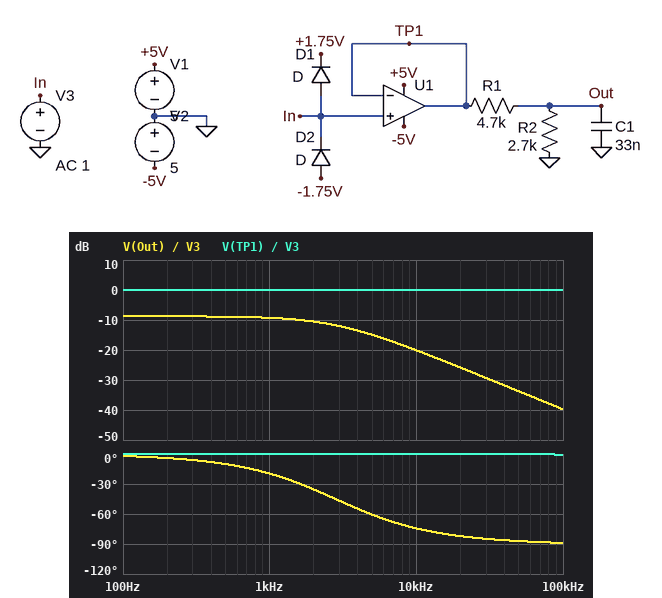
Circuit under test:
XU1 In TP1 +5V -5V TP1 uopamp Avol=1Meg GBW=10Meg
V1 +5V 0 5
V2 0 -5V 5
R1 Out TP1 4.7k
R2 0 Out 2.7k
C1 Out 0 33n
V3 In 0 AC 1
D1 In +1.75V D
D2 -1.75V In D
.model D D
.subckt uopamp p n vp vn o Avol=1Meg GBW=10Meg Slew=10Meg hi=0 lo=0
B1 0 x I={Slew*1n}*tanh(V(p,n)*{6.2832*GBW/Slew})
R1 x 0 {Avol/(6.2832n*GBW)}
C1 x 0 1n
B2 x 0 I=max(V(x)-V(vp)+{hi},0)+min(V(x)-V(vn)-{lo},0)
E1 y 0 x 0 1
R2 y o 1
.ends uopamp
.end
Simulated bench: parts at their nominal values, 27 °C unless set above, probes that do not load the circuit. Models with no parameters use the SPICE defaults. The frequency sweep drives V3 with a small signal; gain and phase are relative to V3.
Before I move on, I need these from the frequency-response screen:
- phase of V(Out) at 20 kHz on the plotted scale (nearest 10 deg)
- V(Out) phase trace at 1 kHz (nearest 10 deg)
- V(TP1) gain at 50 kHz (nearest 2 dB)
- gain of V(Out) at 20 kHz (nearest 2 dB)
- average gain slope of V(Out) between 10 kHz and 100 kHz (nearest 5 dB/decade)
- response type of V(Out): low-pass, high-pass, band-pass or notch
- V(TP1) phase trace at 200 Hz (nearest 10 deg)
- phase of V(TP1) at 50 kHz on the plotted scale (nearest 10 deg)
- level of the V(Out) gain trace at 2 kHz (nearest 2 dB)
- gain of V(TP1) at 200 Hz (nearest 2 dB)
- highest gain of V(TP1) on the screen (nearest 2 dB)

-80 deg
-20 deg
0 dB
-26 dB
-20 dB/decade
low-pass
0 deg
0 deg
-10 dB
0 dB
0 dB
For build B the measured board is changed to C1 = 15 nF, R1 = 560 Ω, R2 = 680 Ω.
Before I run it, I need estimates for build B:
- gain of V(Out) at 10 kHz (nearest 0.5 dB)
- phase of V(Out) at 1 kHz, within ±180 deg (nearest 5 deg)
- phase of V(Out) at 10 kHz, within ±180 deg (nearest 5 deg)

-5.5 dB
0 deg
-15 deg
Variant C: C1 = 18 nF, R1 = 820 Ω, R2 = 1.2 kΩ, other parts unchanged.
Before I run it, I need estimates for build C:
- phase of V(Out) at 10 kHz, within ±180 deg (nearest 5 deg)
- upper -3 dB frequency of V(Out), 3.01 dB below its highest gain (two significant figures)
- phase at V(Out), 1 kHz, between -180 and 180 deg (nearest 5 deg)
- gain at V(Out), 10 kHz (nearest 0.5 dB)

-30 deg
18 kHz
-5 deg
-5.5 dB
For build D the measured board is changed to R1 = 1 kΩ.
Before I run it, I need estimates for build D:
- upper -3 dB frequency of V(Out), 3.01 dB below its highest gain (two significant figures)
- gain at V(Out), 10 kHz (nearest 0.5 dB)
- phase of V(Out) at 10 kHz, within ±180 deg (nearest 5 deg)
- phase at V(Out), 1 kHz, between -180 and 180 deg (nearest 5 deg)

6.6 kHz
-8.0 dB
-55 deg
-10 deg
